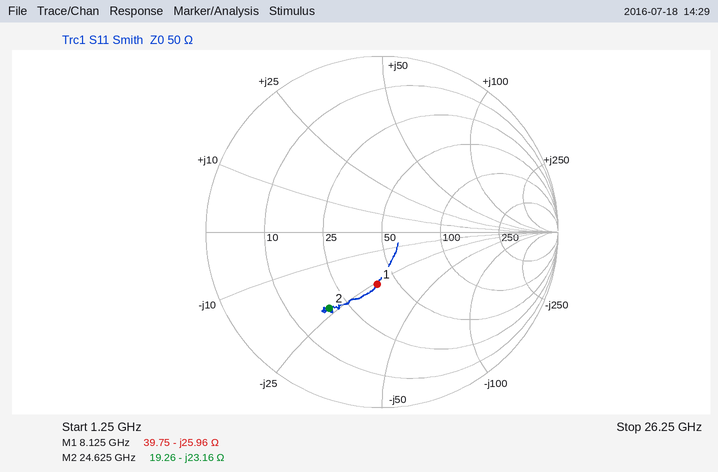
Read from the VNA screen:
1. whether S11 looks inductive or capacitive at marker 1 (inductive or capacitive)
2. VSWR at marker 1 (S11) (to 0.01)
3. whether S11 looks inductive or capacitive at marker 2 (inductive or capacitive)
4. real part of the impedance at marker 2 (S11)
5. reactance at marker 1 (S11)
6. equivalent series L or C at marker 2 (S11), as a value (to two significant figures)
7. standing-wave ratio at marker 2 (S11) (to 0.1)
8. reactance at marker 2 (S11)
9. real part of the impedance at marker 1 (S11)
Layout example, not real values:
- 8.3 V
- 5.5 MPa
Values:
- capacitive
- 1.85
- capacitive
- 19.26 Ω
- -25.96 Ω
- 280 fF
- 3.2
- -23.16 Ω
- 39.75 Ω
